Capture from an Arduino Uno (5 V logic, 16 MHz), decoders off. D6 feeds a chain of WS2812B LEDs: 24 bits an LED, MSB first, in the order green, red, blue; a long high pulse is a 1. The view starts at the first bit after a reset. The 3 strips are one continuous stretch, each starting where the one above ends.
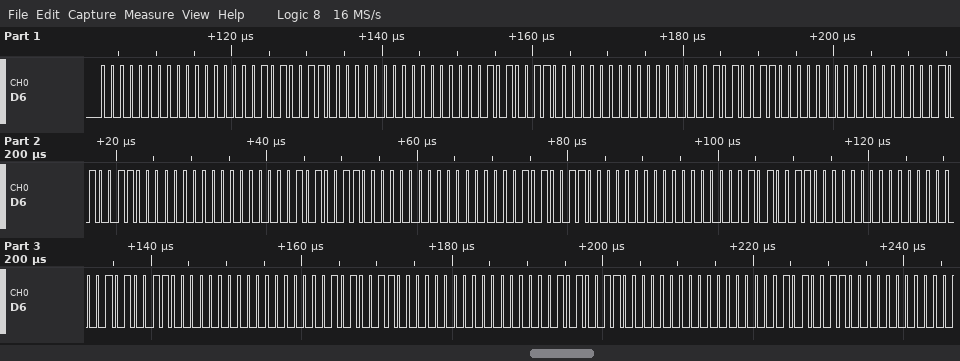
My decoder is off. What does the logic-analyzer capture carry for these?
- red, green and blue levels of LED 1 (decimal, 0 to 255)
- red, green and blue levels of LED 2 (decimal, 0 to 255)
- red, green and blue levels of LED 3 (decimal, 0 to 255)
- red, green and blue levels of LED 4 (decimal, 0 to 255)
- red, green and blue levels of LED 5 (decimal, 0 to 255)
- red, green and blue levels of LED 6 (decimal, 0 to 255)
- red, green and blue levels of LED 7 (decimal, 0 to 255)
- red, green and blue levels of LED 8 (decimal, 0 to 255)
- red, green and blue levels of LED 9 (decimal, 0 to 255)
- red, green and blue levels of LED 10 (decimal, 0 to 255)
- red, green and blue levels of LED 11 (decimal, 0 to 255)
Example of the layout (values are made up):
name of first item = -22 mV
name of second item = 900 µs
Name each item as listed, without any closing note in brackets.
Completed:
red, green and blue levels of LED 1 = 0, 0, 83
red, green and blue levels of LED 2 = 0, 0, 83
red, green and blue levels of LED 3 = 0, 0, 83
red, green and blue levels of LED 4 = 0, 0, 83
red, green and blue levels of LED 5 = 0, 0, 83
red, green and blue levels of LED 6 = 0, 0, 83
red, green and blue levels of LED 7 = 0, 0, 83
red, green and blue levels of LED 8 = 0, 0, 83
red, green and blue levels of LED 9 = 0, 0, 83
red, green and blue levels of LED 10 = 0, 0, 83
red, green and blue levels of LED 11 = 0, 0, 83
